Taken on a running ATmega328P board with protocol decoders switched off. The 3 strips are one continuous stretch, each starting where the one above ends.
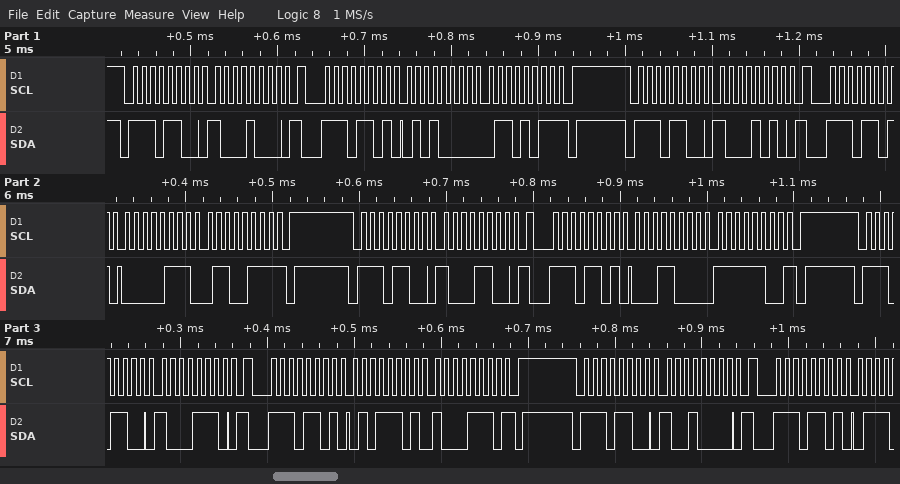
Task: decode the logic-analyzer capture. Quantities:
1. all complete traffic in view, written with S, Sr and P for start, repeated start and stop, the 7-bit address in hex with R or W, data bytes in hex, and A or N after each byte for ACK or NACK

S 76W A 88 A Sr 76R A 50 A 6B N P S 76W A 8A A Sr 76R A 07 A 67 N P S 76W A 8C A Sr 76R A 18 A FC N P S 76W A 8E A Sr 76R A 5D A 8E N P S 76W A 90 A Sr 76R A
